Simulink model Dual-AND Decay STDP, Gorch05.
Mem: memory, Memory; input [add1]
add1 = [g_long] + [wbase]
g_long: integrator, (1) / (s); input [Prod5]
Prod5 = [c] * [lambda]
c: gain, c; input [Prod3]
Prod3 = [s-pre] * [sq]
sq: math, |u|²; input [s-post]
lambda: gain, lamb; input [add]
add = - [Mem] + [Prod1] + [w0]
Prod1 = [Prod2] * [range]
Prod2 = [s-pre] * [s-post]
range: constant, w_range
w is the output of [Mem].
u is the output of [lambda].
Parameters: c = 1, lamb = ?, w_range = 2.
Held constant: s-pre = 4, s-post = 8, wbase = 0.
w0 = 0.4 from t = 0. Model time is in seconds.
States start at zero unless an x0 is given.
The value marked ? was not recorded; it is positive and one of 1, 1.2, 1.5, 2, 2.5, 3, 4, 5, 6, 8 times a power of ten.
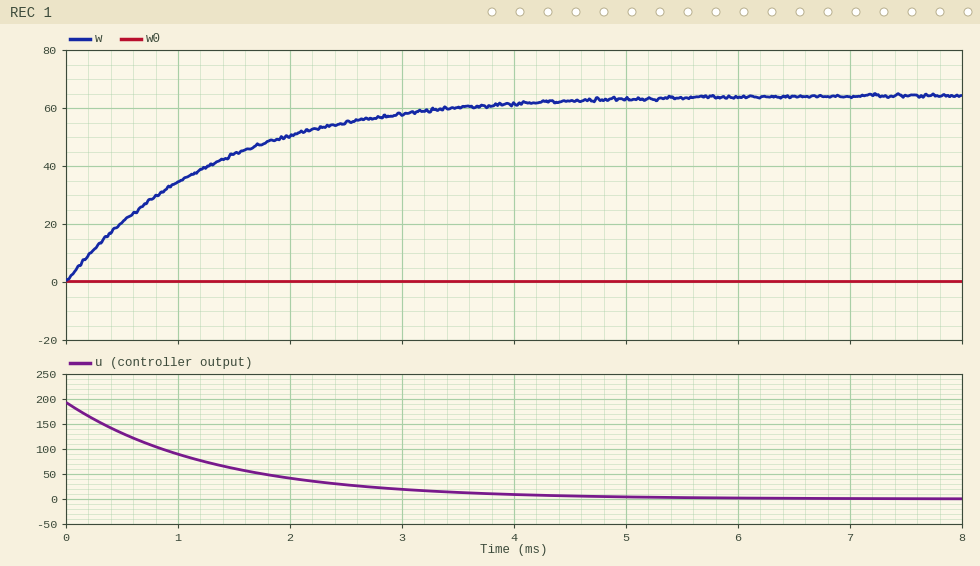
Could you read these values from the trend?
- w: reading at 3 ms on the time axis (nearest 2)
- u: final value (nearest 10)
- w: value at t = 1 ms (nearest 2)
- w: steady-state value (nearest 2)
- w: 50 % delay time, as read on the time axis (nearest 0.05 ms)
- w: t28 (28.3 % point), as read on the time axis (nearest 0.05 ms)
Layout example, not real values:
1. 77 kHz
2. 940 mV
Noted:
1. 58
2. 0
3. 34
4. 64
5. 0.90 ms
6. 0.45 ms
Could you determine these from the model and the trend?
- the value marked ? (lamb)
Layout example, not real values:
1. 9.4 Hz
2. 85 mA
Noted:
1. 3
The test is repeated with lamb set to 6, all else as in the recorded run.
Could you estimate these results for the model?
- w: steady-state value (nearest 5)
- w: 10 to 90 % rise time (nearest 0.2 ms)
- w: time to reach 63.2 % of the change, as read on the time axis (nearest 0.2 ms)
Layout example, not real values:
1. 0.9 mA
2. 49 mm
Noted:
1. 65
2. 1.4 ms
3. 0.6 ms
